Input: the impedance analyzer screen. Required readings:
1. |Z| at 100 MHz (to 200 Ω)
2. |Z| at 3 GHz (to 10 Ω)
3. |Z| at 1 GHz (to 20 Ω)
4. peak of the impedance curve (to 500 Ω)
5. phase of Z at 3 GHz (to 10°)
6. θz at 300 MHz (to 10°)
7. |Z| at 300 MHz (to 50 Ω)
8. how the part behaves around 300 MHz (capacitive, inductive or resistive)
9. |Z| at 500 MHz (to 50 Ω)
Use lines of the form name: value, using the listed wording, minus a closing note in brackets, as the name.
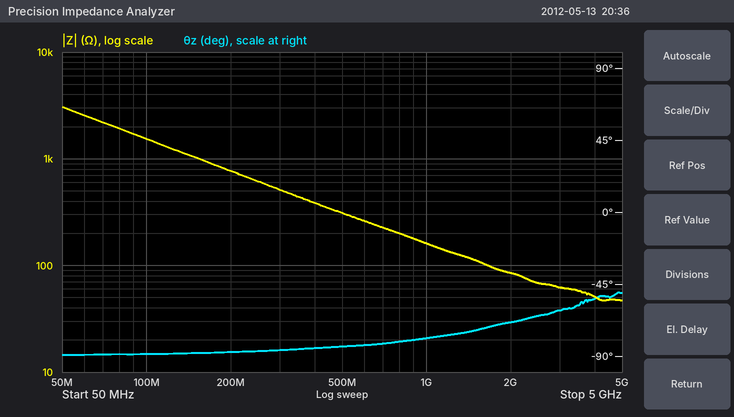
|Z| at 100 MHz: 1.6 kΩ
|Z| at 3 GHz: 60 Ω
|Z| at 1 GHz: 160 Ω
peak of the impedance curve: 3.0 kΩ
phase of Z at 3 GHz: -60°
θz at 300 MHz: -90°
|Z| at 300 MHz: 500 Ω
how the part behaves around 300 MHz: capacitive
|Z| at 500 MHz: 300 Ω
